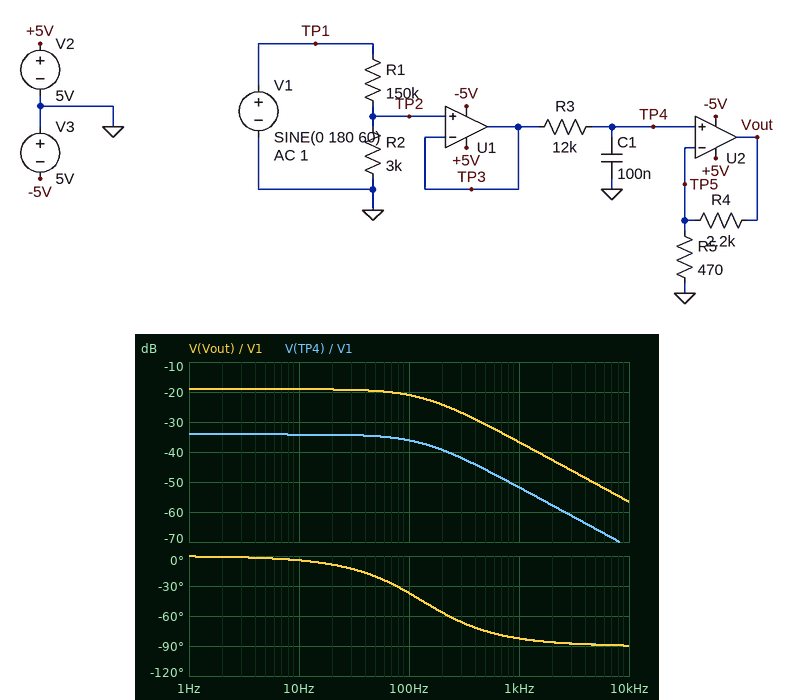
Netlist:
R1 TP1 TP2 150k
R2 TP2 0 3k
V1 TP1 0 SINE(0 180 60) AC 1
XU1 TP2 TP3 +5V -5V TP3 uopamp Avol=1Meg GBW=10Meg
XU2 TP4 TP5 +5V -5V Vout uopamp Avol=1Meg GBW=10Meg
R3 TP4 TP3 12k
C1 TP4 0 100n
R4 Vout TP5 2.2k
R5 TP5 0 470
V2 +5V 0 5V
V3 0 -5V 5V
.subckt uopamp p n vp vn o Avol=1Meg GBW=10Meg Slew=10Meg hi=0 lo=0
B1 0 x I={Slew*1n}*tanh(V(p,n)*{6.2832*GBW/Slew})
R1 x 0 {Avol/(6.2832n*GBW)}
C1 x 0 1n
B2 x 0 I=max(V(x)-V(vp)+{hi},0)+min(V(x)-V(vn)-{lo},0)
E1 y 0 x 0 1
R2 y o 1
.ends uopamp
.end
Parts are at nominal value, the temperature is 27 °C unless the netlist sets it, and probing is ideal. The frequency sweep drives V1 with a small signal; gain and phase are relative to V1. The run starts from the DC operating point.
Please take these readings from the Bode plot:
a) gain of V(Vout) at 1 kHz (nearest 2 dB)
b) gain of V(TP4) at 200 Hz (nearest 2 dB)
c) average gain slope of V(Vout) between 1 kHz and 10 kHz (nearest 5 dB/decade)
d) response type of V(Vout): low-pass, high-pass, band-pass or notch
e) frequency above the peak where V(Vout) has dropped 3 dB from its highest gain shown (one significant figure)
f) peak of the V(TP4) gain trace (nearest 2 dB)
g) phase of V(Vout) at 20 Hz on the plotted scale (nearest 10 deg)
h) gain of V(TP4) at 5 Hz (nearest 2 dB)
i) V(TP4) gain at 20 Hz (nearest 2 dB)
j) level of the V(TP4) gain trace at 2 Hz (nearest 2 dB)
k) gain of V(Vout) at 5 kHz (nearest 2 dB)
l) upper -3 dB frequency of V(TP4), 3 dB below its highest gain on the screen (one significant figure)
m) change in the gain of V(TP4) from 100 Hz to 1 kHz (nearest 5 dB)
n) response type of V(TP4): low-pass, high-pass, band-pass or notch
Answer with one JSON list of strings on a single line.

["-36 dB", "-40 dB", "-20 dB/decade", "low-pass", "100 Hz", "-34 dB", "-10 deg", "-34 dB", "-34 dB", "-34 dB", "-50 dB", "100 Hz", "-15 dB", "low-pass"]
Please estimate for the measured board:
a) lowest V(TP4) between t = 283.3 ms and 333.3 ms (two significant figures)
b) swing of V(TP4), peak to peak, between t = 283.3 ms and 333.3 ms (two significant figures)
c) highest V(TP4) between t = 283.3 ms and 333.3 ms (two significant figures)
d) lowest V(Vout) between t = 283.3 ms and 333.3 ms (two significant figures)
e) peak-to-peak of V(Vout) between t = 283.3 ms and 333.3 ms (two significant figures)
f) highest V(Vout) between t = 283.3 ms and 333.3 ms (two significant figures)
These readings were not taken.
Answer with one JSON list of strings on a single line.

["-3.2 V", "6.4 V", "3.2 V", "-5.0 V", "10 V", "5.0 V"]
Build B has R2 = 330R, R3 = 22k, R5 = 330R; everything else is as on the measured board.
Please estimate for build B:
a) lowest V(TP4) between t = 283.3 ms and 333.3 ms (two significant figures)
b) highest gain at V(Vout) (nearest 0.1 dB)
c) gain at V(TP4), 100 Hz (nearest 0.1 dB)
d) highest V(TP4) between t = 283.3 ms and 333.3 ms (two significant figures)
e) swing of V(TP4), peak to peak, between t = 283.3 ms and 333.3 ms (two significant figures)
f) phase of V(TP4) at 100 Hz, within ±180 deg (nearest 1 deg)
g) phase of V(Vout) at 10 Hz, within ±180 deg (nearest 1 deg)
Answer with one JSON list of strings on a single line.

["-300 mV", "-35.5 dB", "-57.8 dB", "300 mV", "610 mV", "-54 deg", "-8 deg"]
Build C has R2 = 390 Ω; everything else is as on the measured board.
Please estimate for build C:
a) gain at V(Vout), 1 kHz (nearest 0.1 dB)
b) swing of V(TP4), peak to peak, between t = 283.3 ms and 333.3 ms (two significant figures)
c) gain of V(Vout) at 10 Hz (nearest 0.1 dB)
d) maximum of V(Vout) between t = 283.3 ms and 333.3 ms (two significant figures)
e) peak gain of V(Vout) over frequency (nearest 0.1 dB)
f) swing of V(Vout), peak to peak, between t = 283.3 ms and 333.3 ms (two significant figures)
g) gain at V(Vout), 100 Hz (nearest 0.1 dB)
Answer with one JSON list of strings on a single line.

["-54.3 dB", "850 mV", "-36.7 dB", "2.4 V", "-36.6 dB", "4.8 V", "-38.6 dB"]
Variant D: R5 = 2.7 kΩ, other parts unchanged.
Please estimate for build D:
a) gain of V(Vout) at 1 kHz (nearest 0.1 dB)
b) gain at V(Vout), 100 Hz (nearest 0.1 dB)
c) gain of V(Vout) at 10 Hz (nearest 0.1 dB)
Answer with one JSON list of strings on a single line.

["-46.6 dB", "-30.9 dB", "-29.0 dB"]
